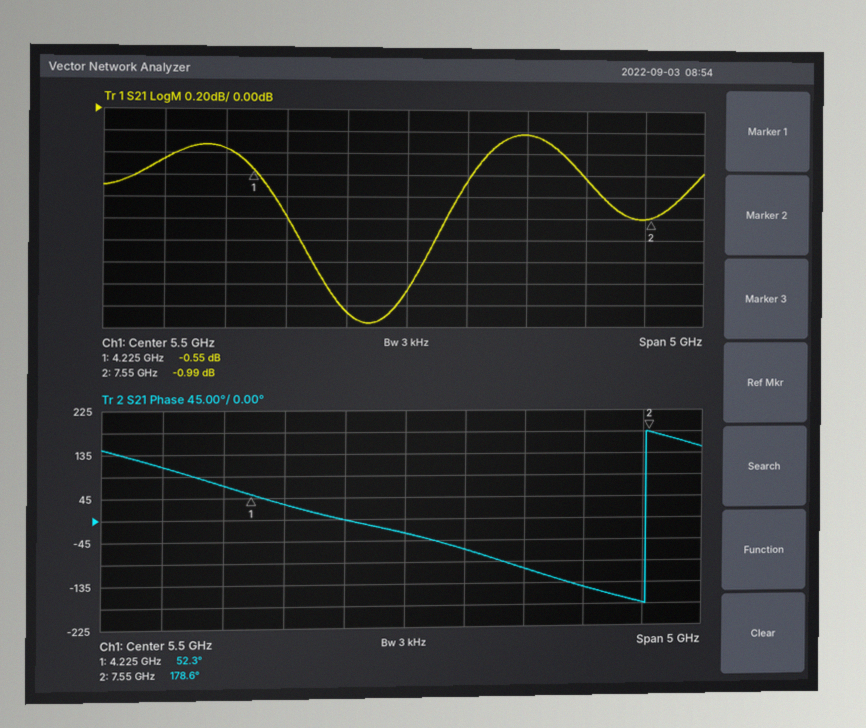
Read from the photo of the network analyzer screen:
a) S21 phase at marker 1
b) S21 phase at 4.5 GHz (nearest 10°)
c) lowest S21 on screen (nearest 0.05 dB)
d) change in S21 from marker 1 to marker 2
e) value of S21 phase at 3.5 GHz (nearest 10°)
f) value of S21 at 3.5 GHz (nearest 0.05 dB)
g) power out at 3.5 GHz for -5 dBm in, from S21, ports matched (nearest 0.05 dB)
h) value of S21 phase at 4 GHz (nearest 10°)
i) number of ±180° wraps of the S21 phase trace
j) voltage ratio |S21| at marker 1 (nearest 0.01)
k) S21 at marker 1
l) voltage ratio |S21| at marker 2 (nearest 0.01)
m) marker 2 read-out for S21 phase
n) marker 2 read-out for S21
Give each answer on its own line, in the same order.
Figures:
52.3°
30°
-1.95 dB
-0.44 dB
110°
-0.45 dB
-5.45 dBm
70°
1
0.94
-0.55 dB
0.89
178.6°
-0.99 dB
